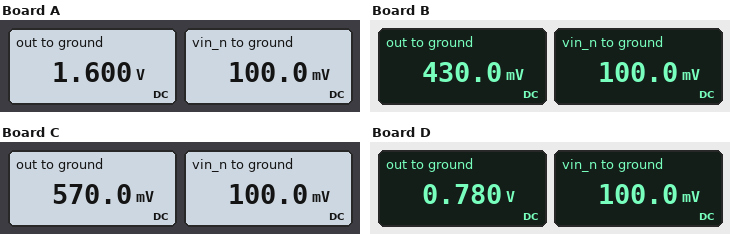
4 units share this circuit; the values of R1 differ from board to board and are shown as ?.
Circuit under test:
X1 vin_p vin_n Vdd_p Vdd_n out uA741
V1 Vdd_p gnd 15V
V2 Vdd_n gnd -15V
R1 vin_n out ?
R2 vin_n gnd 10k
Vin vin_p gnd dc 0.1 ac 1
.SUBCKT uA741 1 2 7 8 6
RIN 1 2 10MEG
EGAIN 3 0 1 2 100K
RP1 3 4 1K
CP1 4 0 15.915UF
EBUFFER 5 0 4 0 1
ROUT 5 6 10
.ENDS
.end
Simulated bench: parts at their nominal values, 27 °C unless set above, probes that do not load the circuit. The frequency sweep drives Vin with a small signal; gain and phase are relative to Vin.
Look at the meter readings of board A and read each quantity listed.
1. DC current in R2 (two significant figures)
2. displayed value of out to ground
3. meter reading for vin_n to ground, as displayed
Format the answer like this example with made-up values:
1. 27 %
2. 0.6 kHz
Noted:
1. 10 µA
2. 1.600 V
3. 100.0 mV
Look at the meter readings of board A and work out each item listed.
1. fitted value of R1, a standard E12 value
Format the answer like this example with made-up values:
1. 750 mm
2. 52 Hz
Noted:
1. 150 kΩ
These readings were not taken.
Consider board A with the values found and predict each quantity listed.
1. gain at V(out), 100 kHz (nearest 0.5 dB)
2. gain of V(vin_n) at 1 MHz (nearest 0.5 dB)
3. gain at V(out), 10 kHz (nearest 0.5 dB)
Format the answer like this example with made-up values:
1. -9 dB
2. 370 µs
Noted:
1. 18.5 dB
2. -24.0 dB
3. 24.0 dB
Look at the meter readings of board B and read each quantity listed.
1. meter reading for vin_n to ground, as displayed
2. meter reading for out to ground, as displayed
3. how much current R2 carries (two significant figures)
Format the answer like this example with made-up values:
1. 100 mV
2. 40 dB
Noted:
1. 100.0 mV
2. 430.0 mV
3. 10 µA
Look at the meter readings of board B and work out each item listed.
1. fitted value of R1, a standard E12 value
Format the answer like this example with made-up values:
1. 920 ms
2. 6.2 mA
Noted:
1. 33 kΩ
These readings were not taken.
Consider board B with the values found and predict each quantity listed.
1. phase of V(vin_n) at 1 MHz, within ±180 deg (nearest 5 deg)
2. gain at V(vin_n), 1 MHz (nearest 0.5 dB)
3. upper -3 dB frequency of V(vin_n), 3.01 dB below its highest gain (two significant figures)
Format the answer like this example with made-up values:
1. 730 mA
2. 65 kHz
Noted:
1. -75 deg
2. -13.0 dB
3. 230 kHz
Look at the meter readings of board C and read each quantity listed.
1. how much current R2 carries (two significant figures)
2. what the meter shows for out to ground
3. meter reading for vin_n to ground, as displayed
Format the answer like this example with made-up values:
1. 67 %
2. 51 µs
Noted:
1. 10 µA
2. 570.0 mV
3. 100.0 mV
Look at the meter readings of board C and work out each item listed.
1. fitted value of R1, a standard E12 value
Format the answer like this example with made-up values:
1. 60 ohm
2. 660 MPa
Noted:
1. 47 kΩ
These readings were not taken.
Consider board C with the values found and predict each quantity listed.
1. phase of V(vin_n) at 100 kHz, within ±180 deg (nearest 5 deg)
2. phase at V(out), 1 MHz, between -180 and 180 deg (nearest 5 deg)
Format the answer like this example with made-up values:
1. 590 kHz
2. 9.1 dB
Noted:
1. -30 deg
2. -80 deg
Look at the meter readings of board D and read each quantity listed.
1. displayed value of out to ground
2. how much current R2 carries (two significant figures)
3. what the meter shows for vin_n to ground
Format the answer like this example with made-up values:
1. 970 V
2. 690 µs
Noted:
1. 0.780 V
2. 10 µA
3. 100.0 mV
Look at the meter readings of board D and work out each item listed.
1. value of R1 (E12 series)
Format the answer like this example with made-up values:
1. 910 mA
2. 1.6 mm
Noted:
1. 68 kΩ
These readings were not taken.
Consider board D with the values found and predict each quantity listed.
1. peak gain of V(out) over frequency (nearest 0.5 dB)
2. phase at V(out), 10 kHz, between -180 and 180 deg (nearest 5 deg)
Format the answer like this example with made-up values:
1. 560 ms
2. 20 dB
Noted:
1. 18.0 dB
2. -5 deg
